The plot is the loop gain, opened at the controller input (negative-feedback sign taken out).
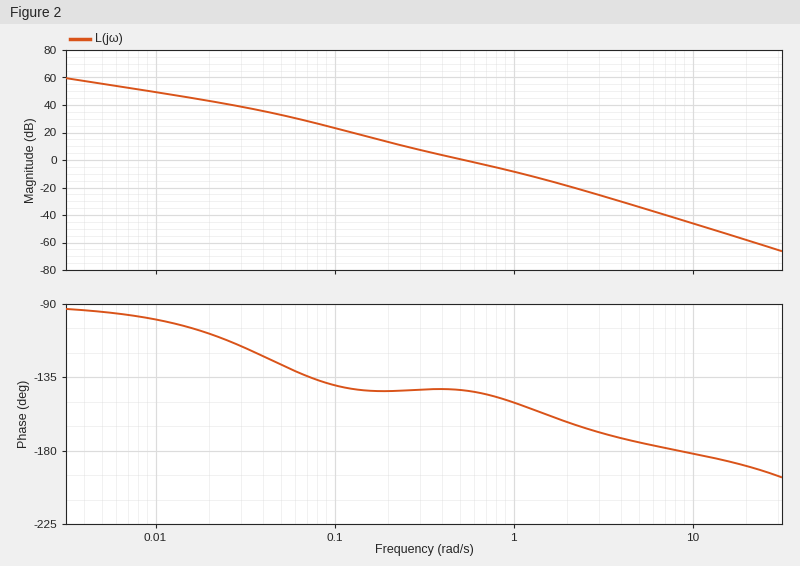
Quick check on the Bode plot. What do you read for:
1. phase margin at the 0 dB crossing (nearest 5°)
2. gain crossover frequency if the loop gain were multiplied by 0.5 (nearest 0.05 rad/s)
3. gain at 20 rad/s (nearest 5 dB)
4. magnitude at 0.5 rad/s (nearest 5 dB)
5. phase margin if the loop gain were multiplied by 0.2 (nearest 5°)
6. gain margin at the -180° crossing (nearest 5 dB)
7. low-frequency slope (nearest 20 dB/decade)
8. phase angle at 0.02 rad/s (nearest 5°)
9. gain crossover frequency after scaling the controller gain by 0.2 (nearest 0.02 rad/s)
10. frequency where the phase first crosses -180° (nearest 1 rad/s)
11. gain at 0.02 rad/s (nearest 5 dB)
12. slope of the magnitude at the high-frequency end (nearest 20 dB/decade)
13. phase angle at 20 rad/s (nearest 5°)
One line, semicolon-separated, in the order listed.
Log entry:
35°; 0.35 rad/s; -60 dB; 0 dB; 35°; 45 dB; -20 dB/decade; -110°; 0.18 rad/s; 8 rad/s; 45 dB; -40 dB/decade; -190°
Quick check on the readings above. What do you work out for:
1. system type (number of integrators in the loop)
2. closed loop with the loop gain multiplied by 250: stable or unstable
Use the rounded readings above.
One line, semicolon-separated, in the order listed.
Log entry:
1; unstable
